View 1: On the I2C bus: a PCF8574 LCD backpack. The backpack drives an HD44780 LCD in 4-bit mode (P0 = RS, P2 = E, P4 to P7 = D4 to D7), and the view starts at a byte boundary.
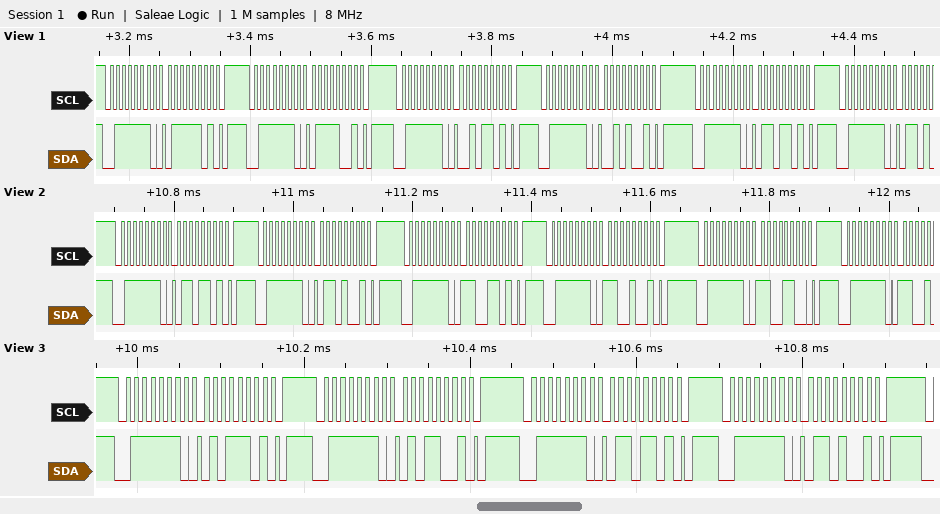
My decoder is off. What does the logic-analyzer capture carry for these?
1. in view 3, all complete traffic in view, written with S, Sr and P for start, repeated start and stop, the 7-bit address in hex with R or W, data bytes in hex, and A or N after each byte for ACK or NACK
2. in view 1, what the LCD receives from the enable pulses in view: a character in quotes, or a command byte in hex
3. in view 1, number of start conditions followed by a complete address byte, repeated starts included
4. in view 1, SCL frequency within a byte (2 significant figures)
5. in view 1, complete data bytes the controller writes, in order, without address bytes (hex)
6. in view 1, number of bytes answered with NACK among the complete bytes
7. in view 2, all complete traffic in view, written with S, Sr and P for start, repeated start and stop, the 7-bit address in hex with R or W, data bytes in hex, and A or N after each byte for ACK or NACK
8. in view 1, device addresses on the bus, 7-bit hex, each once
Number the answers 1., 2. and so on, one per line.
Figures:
1. S 3FW A 5D A P S 3FW A 59 A P S 3FW A 6D A P S 3FW A 69 A P
2. 'r'
3. 6
4. 100 kHz
5. 7D 79 2D 29 6D
6. 0
7. S 3FW A 6D A P S 3FW A 69 A P S 3FW A CD A P S 3FW A C9 A P S 3FW A CC A P S 3FW A
8. 0x3F
